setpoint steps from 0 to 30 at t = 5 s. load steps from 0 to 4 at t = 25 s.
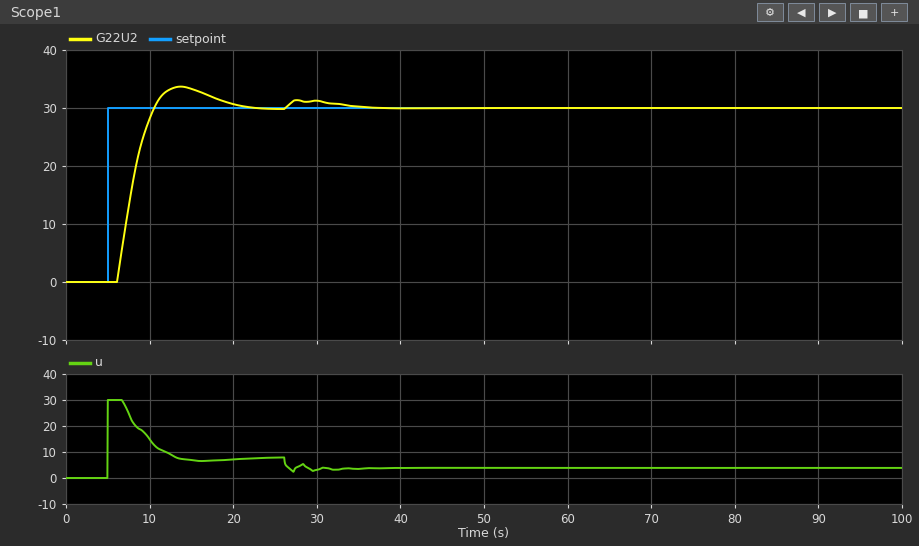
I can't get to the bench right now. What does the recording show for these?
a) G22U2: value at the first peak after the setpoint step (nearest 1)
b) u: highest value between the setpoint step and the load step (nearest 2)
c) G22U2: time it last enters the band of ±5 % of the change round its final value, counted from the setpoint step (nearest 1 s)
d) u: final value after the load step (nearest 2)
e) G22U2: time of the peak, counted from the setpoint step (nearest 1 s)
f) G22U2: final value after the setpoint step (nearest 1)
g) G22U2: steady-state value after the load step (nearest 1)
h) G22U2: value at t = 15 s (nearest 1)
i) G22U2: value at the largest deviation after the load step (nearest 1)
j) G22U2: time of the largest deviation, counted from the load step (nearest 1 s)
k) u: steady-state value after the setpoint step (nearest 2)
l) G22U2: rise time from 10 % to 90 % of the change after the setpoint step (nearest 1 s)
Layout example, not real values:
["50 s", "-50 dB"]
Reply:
["34", "30", "13 s", "4", "9 s", "30", "30", "33", "31", "3 s", "8", "3 s"]
